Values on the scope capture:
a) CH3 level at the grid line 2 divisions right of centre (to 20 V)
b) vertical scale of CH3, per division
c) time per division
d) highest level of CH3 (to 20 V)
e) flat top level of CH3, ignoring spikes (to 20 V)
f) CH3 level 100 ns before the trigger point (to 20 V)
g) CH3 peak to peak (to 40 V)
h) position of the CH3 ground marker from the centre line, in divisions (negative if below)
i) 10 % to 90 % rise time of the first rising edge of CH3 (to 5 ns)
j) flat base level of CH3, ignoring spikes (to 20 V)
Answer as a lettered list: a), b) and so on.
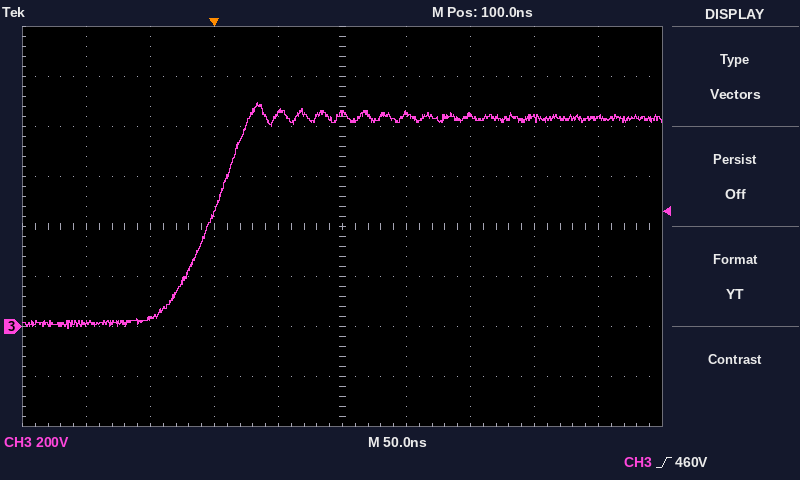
a) 840 V
b) 200 V
c) 50 ns
d) 900 V
e) 840 V
f) 20 V
g) 920 V
h) -2.0 div
i) 55 ns
j) 20 V
